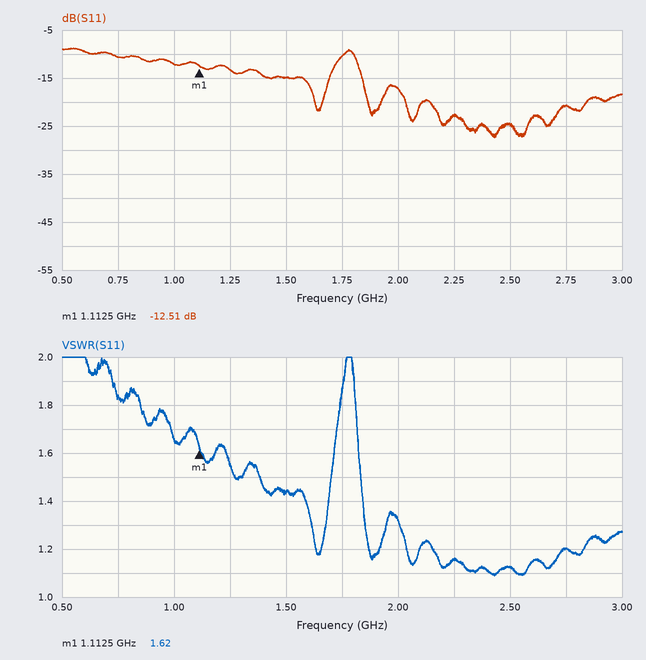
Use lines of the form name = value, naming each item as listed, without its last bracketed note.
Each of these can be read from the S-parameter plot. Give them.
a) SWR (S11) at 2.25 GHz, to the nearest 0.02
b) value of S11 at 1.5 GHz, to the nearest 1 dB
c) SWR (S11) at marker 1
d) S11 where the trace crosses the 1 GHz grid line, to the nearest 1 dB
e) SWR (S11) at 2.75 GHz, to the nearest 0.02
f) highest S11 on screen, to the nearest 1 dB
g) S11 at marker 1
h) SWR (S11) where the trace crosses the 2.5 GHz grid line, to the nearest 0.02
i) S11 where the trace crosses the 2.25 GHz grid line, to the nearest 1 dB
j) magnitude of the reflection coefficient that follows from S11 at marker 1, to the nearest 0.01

SWR (S11) at 2.25 GHz, to the nearest 0.02 = 1.16
value of S11 at 1.5 GHz, to the nearest 1 dB = -15 dB
SWR (S11) at marker 1 = 1.62
S11 where the trace crosses the 1 GHz grid line, to the nearest 1 dB = -12 dB
SWR (S11) at 2.75 GHz, to the nearest 0.02 = 1.20
highest S11 on screen, to the nearest 1 dB = -9 dB
S11 at marker 1 = -12.51 dB
SWR (S11) where the trace crosses the 2.5 GHz grid line, to the nearest 0.02 = 1.12
S11 where the trace crosses the 2.25 GHz grid line, to the nearest 1 dB = -23 dB
magnitude of the reflection coefficient that follows from S11 at marker 1, to the nearest 0.01 = 0.24
